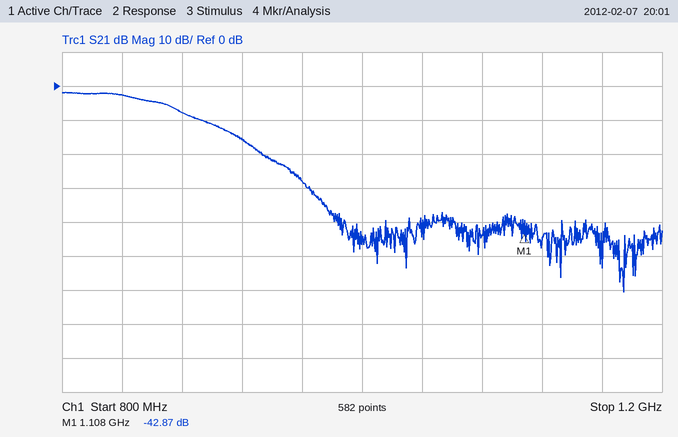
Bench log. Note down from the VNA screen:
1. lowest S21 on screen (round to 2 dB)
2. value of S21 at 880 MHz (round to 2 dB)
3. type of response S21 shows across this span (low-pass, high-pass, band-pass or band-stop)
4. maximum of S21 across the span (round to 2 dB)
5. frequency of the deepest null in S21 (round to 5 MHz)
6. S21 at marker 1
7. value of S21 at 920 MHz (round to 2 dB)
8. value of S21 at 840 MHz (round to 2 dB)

-60 dB
-8 dB
low-pass
-2 dB
1.175 GHz
-42.87 dB
-16 dB
-2 dB
